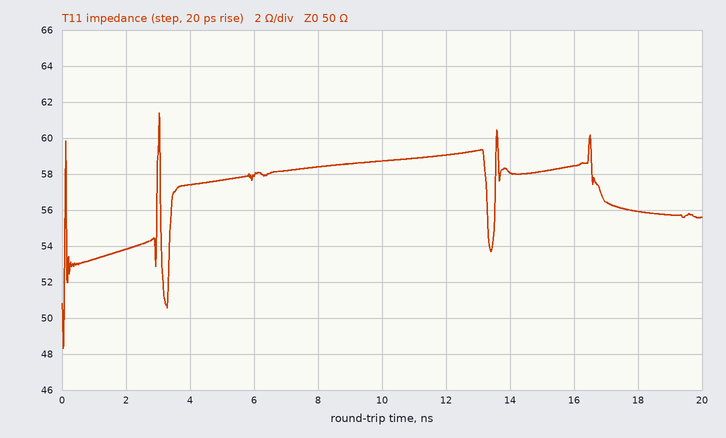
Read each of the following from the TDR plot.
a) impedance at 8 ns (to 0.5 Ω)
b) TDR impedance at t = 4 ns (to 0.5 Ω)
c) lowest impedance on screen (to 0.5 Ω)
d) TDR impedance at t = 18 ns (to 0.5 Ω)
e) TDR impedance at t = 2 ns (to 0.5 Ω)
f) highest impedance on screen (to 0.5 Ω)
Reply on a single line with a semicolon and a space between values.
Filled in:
58.5 Ω; 57.5 Ω; 48.5 Ω; 56.0 Ω; 54.0 Ω; 61.5 Ω
